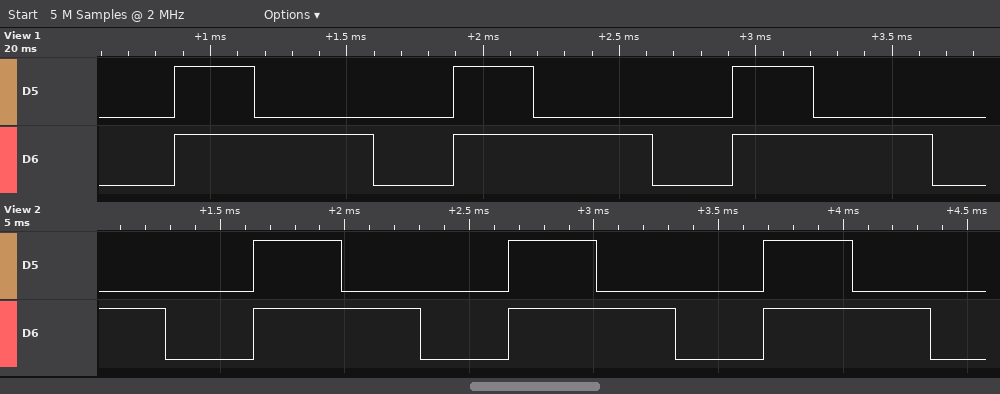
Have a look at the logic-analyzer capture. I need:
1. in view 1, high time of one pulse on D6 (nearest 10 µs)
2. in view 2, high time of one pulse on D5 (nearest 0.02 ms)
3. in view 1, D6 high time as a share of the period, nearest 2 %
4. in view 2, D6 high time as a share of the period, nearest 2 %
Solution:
730 µs
0.36 ms
72 %
66 %
